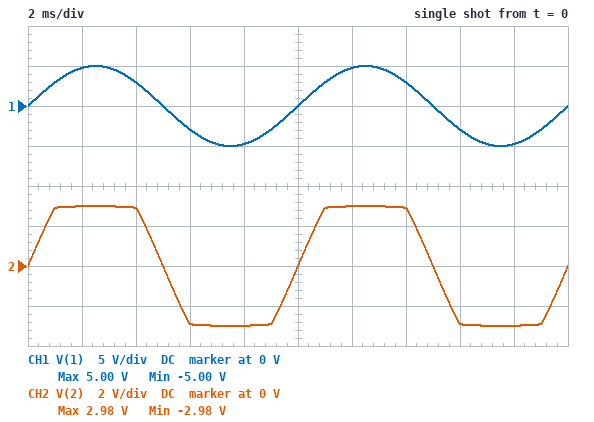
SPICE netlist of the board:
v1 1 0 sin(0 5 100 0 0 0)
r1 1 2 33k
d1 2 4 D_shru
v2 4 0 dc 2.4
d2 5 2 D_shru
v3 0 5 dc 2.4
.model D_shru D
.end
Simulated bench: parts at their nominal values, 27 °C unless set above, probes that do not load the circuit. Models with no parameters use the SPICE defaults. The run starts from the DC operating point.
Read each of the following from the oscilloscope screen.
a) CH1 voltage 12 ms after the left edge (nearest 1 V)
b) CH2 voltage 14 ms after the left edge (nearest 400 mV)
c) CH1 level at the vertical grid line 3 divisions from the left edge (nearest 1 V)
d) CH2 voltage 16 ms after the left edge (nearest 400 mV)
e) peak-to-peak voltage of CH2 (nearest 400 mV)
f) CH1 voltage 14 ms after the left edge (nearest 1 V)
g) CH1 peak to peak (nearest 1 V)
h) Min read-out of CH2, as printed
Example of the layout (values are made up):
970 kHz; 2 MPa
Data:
5 V; 2.8 V; -3 V; -2.8 V; 6.0 V; 3 V; 10 V; -2.98 V
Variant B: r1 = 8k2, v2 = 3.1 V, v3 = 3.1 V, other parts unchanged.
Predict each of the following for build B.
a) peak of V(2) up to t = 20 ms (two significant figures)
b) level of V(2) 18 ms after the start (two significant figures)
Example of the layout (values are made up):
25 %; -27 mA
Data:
3.7 V; -3.7 V
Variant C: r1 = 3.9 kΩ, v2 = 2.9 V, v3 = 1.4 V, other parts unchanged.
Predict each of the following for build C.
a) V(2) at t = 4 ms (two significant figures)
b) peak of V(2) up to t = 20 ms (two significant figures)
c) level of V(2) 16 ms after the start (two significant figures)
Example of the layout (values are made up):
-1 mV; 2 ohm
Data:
2.9 V; 3.5 V; -2.0 V
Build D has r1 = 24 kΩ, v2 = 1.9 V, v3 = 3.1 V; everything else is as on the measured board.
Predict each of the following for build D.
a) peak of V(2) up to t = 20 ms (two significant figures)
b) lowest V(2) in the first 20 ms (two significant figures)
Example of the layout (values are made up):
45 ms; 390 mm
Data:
2.5 V; -3.7 V
